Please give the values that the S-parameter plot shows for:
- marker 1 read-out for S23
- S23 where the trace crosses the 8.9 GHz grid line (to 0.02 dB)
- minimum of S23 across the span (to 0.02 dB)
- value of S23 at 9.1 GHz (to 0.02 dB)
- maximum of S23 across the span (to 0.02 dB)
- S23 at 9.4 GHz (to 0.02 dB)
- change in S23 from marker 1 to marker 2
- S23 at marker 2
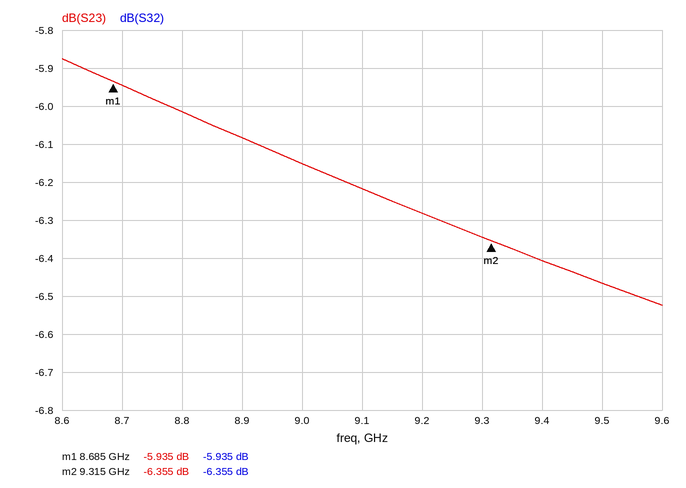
-5.935 dB
-6.08 dB
-6.52 dB
-6.22 dB
-5.88 dB
-6.40 dB
-0.420 dB
-6.355 dB
